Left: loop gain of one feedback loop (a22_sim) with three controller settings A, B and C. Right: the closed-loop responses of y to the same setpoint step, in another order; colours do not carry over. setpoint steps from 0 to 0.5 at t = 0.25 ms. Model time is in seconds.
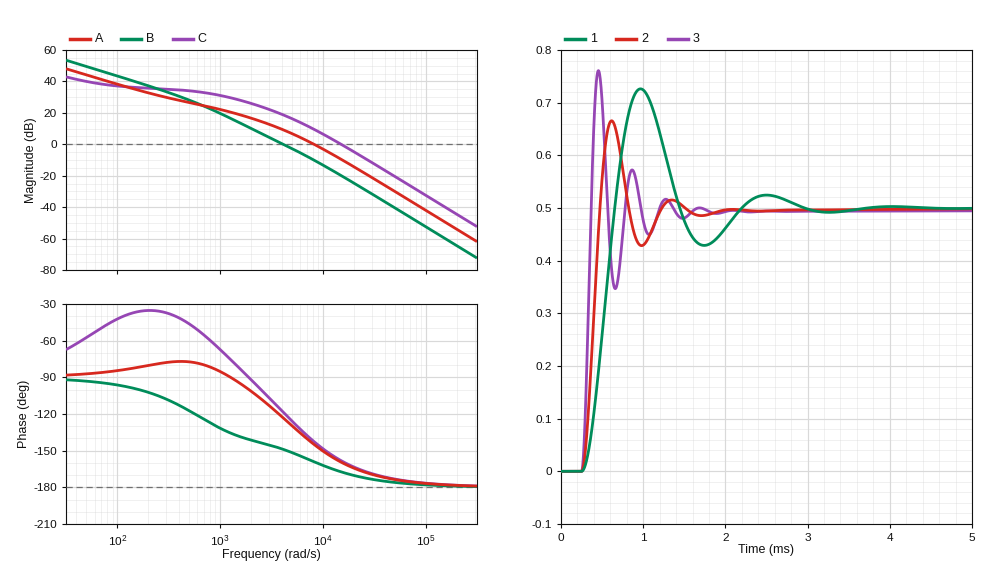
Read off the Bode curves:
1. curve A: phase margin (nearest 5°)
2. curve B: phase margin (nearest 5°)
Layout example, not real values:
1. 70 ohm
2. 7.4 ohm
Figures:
1. 35°
2. 30°
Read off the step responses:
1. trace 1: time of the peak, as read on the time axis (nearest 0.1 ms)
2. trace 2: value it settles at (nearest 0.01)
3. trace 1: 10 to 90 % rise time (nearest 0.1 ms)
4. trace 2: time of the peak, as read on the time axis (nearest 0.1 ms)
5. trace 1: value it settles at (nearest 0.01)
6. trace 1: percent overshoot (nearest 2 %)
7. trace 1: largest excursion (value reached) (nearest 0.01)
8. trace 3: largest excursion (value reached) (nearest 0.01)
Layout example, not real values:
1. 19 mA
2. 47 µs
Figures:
1. 1.0 ms
2. 0.50
3. 0.3 ms
4. 0.6 ms
5. 0.50
6. 46 %
7. 0.73
8. 0.76
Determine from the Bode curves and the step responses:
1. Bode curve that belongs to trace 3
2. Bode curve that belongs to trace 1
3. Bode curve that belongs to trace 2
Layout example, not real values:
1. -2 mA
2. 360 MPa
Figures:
1. C
2. B
3. A
